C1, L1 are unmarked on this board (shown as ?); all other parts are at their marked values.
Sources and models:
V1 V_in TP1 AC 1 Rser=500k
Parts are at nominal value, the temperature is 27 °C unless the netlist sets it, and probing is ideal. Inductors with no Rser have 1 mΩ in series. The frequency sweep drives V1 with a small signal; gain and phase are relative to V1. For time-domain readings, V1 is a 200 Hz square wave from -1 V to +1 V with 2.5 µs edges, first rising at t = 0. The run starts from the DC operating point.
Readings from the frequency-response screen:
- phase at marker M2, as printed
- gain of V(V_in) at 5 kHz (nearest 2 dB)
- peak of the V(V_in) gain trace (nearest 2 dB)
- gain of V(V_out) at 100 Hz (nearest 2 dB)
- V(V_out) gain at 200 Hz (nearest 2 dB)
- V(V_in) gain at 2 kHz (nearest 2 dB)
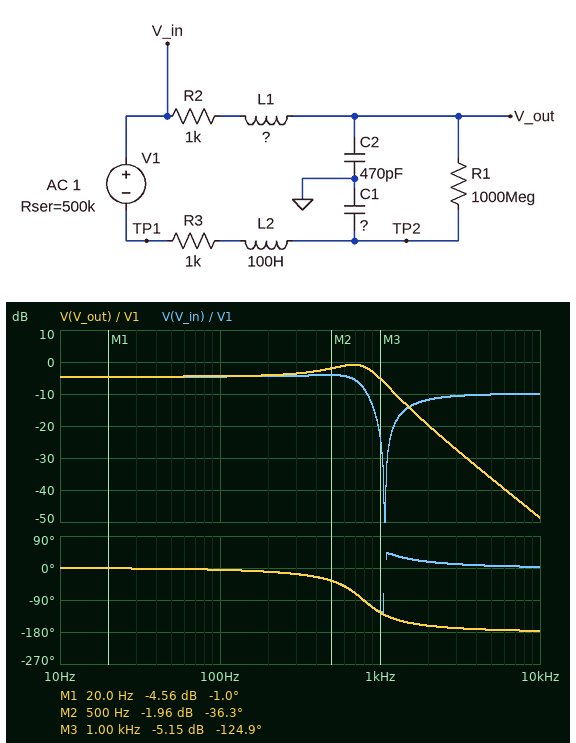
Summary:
-36.3 deg
-10 dB
-4 dB
-4 dB
-4 dB
-12 dB
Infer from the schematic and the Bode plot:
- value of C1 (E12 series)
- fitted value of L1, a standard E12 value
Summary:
680 pF
47 H
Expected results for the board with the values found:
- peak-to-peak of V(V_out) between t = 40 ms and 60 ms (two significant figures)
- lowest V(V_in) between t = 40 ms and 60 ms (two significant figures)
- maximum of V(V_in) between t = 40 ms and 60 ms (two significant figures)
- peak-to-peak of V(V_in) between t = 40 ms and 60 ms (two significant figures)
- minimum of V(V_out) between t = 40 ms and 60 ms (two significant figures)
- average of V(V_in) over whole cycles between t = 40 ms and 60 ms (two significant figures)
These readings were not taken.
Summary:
1.9 V
-710 mV
890 mV
1.6 V
-870 mV
91 mV
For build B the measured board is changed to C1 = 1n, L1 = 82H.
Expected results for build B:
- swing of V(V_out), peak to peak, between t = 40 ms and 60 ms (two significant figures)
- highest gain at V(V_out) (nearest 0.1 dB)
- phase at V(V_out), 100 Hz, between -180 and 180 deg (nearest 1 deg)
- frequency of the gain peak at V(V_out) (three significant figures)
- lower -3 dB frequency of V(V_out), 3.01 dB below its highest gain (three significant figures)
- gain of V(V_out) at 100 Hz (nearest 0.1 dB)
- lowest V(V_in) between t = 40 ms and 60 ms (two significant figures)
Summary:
2.3 V
0.7 dB
-6 deg
582 Hz
256 Hz
-3.2 dB
-730 mV
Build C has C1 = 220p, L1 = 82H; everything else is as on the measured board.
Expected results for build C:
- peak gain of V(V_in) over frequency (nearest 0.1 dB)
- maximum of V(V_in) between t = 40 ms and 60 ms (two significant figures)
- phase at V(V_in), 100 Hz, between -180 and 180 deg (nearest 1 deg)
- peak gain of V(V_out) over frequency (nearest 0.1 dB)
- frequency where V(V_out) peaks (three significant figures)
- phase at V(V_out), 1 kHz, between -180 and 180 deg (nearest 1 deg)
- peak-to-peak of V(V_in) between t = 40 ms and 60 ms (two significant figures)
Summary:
-6.2 dB
410 mV
-3 deg
-2.9 dB
912 Hz
-99 deg
1.2 V
